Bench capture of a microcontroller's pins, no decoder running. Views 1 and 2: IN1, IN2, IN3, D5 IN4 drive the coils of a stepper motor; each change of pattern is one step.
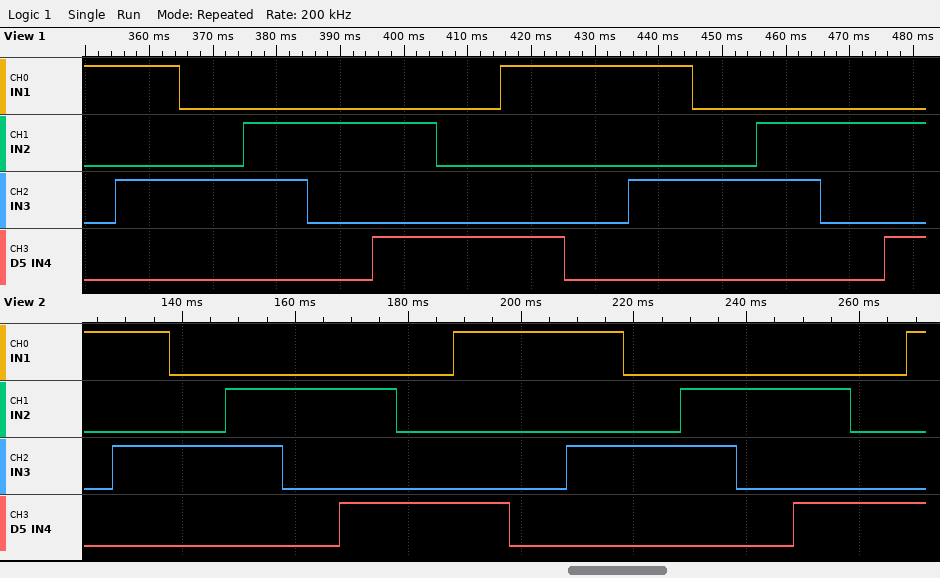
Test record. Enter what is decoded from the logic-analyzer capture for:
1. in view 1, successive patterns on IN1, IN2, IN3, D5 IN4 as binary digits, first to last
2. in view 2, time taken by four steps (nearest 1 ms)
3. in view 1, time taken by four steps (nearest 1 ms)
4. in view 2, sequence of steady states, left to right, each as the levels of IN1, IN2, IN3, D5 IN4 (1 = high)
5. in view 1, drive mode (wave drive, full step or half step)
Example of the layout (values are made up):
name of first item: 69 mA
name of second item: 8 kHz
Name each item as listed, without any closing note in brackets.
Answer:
in view 1, successive patterns on IN1, IN2, IN3, D5 IN4 as binary digits, first to last: 1000 1010 0010 0110 0100 0101 0001 1001 1000 1010 0010 0110 0100 0101
in view 2, time taken by four steps: 40 ms
in view 1, time taken by four steps: 40 ms
in view 2, sequence of steady states, left to right, each as the levels of IN1, IN2, IN3, D5 IN4: 1000 1010 0010 0110 0100 0101 0001 1001 1000 1010 0010 0110 0100 0101 0001 1001
in view 1, drive mode: half step
